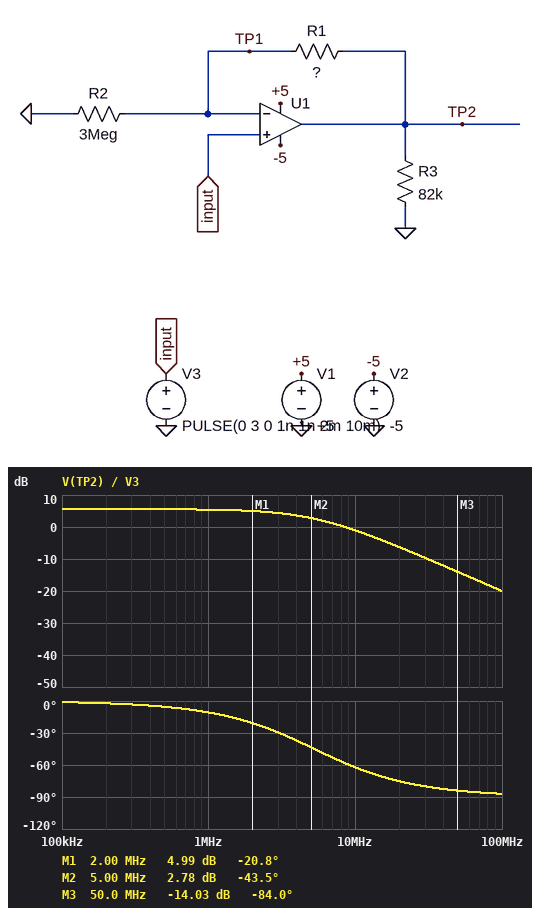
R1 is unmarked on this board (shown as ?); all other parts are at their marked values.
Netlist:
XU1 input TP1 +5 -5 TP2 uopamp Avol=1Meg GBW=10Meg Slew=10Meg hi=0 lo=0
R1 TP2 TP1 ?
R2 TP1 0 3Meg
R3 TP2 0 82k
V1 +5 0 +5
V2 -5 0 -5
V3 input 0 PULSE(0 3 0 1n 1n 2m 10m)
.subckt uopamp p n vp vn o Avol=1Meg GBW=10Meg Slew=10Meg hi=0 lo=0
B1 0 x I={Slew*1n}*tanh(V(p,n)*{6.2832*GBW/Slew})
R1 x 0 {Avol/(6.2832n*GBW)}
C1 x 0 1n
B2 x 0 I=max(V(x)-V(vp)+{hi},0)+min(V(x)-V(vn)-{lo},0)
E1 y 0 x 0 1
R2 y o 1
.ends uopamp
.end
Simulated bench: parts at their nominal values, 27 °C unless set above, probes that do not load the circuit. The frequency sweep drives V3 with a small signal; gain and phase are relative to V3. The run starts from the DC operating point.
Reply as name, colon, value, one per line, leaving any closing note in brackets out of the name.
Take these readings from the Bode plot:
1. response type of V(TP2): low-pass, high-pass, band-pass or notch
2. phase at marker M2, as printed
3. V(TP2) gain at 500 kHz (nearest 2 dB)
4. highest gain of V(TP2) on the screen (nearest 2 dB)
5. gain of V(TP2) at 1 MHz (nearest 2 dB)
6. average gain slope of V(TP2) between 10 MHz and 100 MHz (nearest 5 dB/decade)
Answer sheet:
response type of V(TP2): low-pass, high-pass, band-pass or notch: low-pass
phase at marker M2, as printed: -43.5 deg
V(TP2) gain at 500 kHz: 6 dB
highest gain of V(TP2) on the screen: 6 dB
gain of V(TP2) at 1 MHz: 6 dB
average gain slope of V(TP2) between 10 MHz and 100 MHz: -20 dB/decade
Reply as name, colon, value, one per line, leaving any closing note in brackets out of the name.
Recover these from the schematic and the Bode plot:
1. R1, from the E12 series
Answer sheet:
R1, from the E12 series: 2.7 MΩ
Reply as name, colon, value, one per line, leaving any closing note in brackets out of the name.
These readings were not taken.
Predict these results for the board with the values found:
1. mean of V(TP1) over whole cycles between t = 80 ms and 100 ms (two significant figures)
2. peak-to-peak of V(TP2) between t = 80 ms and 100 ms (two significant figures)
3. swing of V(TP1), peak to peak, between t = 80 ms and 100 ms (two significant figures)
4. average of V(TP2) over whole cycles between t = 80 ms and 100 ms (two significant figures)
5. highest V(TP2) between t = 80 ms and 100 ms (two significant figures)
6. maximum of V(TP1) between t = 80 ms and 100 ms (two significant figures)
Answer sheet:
mean of V(TP1) over whole cycles between t = 80 ms and 100 ms: 530 mV
peak-to-peak of V(TP2) between t = 80 ms and 100 ms: 5.0 V
swing of V(TP1), peak to peak, between t = 80 ms and 100 ms: 2.6 V
average of V(TP2) over whole cycles between t = 80 ms and 100 ms: 1.0 V
highest V(TP2) between t = 80 ms and 100 ms: 5.0 V
maximum of V(TP1) between t = 80 ms and 100 ms: 2.6 V
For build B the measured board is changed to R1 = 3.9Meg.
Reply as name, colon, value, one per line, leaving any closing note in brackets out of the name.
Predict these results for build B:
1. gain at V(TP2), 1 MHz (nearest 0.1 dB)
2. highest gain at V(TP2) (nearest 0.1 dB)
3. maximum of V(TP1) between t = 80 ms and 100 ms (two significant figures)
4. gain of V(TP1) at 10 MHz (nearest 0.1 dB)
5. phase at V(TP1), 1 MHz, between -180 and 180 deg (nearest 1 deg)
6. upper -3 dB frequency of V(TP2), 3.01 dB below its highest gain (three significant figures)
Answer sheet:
gain at V(TP2), 1 MHz: 7.0 dB
highest gain at V(TP2): 7.2 dB
maximum of V(TP1) between t = 80 ms and 100 ms: 2.2 V
gain of V(TP1) at 10 MHz: -8.0 dB
phase at V(TP1), 1 MHz, between -180 and 180 deg: -13 deg
upper -3 dB frequency of V(TP2), 3.01 dB below its highest gain: 4.35 MHz
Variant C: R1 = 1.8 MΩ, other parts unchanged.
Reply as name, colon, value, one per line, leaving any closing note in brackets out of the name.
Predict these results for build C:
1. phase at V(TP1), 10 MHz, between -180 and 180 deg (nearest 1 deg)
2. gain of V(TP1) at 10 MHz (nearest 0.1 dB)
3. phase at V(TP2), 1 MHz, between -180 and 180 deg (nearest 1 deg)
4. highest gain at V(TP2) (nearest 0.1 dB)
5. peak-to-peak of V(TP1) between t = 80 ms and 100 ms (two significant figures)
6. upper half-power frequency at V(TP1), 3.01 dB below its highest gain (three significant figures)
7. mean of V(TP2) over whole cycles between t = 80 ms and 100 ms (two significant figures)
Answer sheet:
phase at V(TP1), 10 MHz, between -180 and 180 deg: -58 deg
gain of V(TP1) at 10 MHz: -5.5 dB
phase at V(TP2), 1 MHz, between -180 and 180 deg: -9 deg
highest gain at V(TP2): 4.1 dB
peak-to-peak of V(TP1) between t = 80 ms and 100 ms: 3.0 V
upper half-power frequency at V(TP1), 3.01 dB below its highest gain: 6.25 MHz
mean of V(TP2) over whole cycles between t = 80 ms and 100 ms: 960 mV
